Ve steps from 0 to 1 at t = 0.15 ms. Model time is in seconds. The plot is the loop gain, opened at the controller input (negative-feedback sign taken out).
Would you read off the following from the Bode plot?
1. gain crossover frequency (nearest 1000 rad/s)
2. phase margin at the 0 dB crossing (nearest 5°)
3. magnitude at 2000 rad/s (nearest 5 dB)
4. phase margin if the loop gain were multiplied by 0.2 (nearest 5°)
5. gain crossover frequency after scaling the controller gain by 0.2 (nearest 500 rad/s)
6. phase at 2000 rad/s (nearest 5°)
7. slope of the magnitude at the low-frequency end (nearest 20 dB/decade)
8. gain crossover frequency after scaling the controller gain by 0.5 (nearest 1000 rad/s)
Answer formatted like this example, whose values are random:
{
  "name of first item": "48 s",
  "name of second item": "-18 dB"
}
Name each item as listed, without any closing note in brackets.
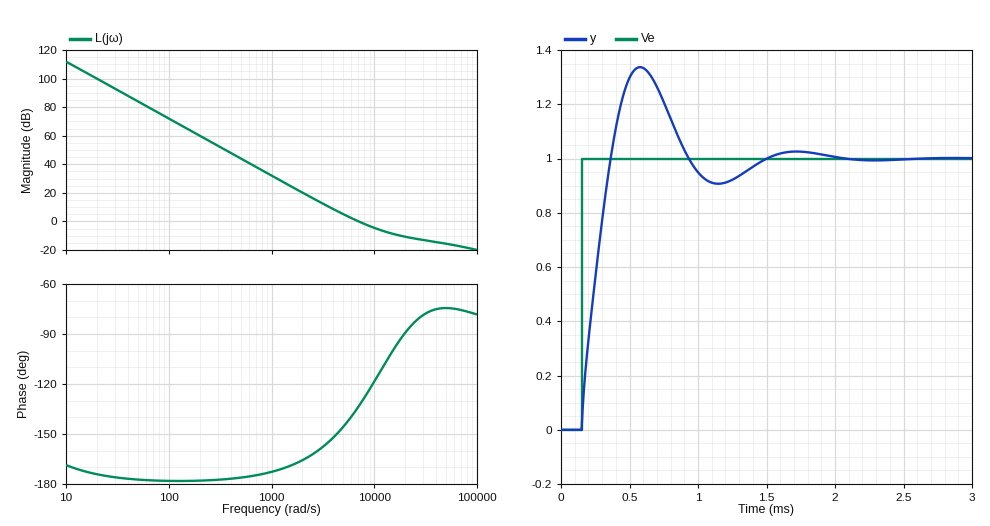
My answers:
{
  "gain crossover frequency": "7000 rad/s",
  "phase margin at the 0 dB crossing": "45°",
  "magnitude at 2000 rad/s": "20 dB",
  "phase margin if the loop gain were multiplied by 0.2": "20°",
  "gain crossover frequency after scaling the controller gain by 0.2": "3000 rad/s",
  "phase at 2000 rad/s": "-165°",
  "slope of the magnitude at the low-frequency end": "-40 dB/decade",
  "gain crossover frequency after scaling the controller gain by 0.5": "5000 rad/s"
}
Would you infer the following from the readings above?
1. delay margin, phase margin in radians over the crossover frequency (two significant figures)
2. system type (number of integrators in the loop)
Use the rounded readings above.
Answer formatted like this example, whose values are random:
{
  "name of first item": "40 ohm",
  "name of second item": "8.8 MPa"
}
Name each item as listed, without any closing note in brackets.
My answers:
{
  "delay margin, phase margin in radians over the crossover frequency": "0.00011 s",
  "system type": "2"
}
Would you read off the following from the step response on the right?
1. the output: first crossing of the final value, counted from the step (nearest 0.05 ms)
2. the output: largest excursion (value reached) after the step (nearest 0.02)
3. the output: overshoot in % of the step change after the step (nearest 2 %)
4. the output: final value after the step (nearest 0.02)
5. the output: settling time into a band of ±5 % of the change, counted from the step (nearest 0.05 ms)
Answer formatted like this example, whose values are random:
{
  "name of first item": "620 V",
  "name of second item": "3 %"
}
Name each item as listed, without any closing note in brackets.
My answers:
{
  "the output: first crossing of the final value, counted from the step": "0.20 ms",
  "the output: largest excursion (value reached) after the step": "1.34",
  "the output: overshoot in % of the step change after the step": "34 %",
  "the output: final value after the step": "1.00",
  "the output: settling time into a band of ±5 % of the change, counted from the step": "1.20 ms"
}
